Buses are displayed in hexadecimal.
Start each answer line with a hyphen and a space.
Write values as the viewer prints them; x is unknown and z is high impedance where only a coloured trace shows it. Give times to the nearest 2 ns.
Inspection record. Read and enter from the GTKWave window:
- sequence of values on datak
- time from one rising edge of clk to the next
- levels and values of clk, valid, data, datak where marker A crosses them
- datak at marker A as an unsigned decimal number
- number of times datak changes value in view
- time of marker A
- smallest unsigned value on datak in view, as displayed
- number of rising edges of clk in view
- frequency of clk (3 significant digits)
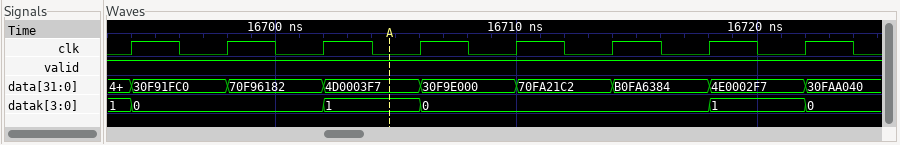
- 1, 0, 1, 0, 1, 0
- 4 ns
- clk=0, valid=1, data=4D0003F7, datak=1
- 1
- 5
- 16704 ns
- 0
- 8
- 250 MHz
